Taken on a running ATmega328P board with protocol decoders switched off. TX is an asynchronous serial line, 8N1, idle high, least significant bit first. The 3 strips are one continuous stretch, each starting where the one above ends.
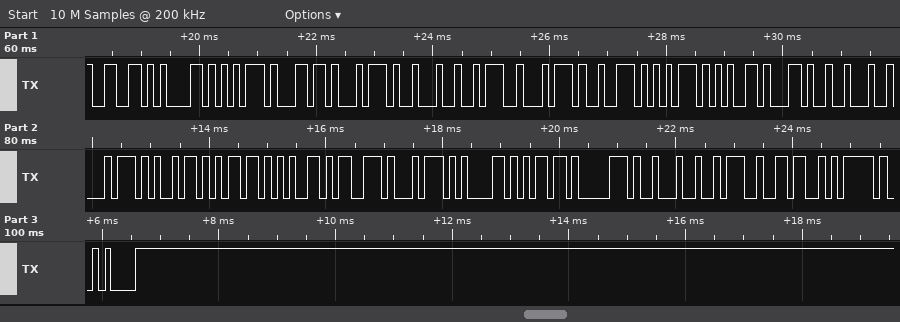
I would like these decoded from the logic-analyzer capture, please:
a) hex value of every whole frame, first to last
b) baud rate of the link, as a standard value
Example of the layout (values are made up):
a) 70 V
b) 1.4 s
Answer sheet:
a) 66 61 75 6C 74 22 3A 74 72 75 65 2C 22 74 69 6D 65 73 74 61 6D 70 22 3A 36 7D 0A
b) 9600 baud
